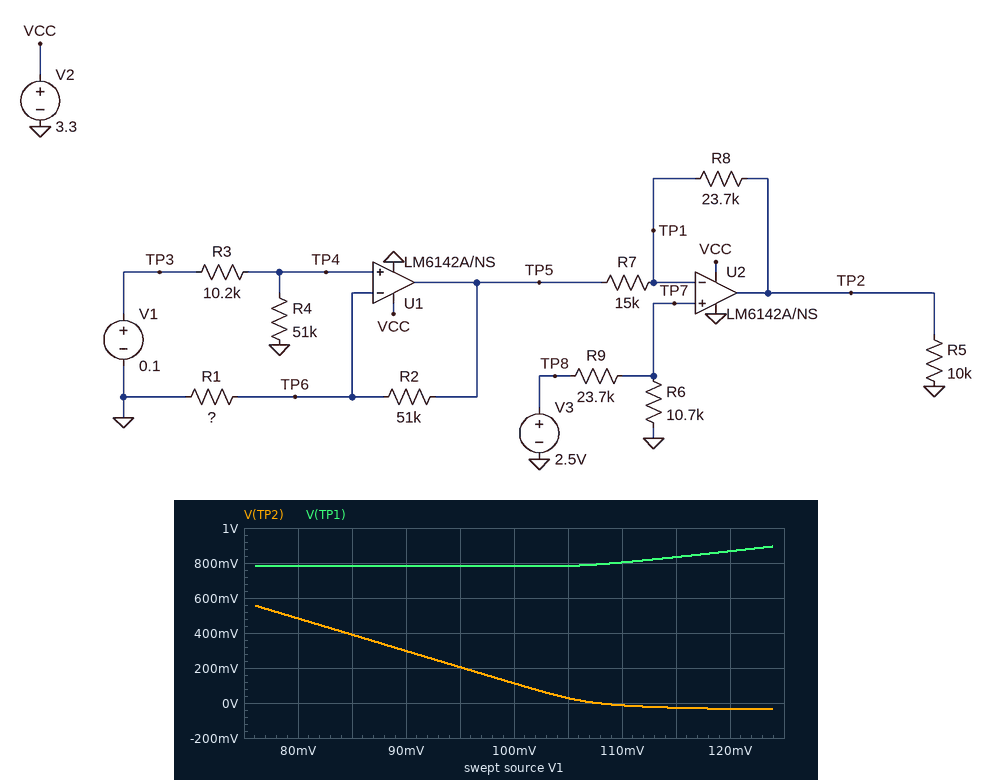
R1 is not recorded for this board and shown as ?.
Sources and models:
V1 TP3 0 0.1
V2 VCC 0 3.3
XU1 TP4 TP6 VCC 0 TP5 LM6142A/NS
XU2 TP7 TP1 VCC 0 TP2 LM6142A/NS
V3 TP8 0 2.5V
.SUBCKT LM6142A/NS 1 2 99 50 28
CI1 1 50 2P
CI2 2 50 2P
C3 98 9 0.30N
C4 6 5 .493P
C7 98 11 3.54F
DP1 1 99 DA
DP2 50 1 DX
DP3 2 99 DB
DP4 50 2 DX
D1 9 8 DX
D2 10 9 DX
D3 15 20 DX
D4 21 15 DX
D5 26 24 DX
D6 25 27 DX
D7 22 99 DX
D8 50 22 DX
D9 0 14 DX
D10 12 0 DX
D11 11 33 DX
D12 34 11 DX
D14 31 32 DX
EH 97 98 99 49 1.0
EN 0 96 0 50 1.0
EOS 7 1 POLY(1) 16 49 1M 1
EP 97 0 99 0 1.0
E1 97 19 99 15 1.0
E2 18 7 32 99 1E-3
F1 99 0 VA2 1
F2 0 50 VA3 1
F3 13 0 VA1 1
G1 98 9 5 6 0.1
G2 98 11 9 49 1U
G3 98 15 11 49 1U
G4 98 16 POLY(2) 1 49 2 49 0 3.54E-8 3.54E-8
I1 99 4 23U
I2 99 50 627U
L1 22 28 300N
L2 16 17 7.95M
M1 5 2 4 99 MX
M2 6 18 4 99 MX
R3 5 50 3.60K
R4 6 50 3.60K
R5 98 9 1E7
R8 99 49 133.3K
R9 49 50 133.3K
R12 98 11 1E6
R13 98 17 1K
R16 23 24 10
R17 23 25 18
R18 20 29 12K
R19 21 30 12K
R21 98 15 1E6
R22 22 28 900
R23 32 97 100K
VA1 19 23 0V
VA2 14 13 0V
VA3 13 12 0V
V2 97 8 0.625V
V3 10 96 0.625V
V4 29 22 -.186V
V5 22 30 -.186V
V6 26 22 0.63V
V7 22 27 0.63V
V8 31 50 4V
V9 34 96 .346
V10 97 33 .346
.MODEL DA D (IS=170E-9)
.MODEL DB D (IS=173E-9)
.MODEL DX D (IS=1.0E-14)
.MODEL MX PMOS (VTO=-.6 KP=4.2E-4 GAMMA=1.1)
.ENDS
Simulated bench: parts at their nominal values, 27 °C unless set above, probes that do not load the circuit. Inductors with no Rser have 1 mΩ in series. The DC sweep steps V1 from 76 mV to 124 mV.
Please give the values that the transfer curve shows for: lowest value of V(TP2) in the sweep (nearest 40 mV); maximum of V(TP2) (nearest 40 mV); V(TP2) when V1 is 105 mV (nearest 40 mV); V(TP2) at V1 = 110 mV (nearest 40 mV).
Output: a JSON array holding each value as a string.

["-40 mV", "560 mV", "40 mV", "0 V"]
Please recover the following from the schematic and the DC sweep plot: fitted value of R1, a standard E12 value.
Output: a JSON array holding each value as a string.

["3.9 kΩ"]
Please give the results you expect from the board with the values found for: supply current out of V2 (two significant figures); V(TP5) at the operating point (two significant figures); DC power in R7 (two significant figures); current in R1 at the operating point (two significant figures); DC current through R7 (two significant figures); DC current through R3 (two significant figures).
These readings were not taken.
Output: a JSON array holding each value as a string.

["1.4 mA", "1.2 V", "12 µW", "22 µA", "28 µA", "1.5 µA"]
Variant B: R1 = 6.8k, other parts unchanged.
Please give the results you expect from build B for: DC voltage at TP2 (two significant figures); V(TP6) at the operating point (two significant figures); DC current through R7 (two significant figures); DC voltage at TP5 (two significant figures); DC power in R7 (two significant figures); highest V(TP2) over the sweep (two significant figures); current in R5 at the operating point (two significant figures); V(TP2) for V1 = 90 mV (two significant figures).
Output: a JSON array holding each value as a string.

["870 mV", "86 mV", "3.9 µA", "720 mV", "230 nW", "1.1 V", "87 µA", "980 mV"]
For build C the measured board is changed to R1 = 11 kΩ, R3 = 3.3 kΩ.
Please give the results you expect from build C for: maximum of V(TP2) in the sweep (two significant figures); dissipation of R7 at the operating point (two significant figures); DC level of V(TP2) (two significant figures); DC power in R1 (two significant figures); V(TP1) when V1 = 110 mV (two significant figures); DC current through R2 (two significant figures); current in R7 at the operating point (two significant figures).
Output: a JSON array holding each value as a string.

["1.4 V", "4.2 µW", "1.2 V", "830 nW", "780 mV", "8.5 µA", "17 µA"]
